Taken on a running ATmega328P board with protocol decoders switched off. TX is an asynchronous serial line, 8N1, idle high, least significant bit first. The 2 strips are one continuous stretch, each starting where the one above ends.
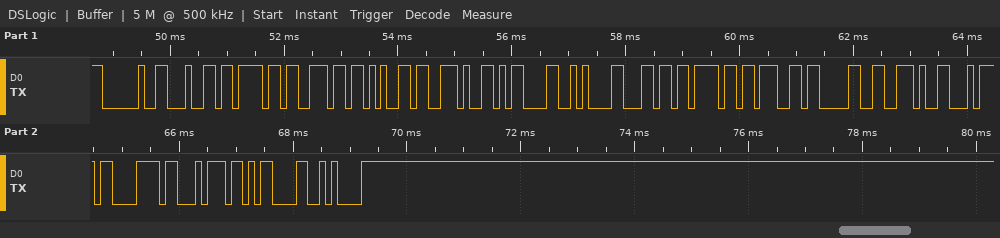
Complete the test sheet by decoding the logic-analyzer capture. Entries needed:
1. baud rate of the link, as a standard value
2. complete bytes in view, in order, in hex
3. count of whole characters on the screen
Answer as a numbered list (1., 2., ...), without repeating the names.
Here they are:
1. 9600 baud
2. 20 64 6F 6E 65 2E 0D 0A 6C 6F 67 30 2E 74 78 74 0D 0A
3. 18
